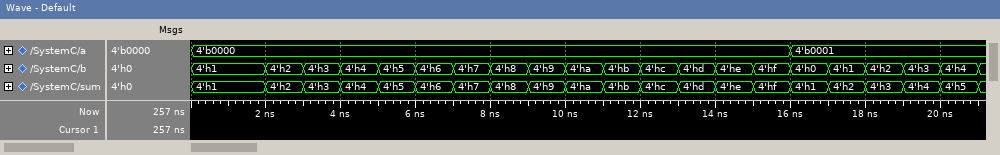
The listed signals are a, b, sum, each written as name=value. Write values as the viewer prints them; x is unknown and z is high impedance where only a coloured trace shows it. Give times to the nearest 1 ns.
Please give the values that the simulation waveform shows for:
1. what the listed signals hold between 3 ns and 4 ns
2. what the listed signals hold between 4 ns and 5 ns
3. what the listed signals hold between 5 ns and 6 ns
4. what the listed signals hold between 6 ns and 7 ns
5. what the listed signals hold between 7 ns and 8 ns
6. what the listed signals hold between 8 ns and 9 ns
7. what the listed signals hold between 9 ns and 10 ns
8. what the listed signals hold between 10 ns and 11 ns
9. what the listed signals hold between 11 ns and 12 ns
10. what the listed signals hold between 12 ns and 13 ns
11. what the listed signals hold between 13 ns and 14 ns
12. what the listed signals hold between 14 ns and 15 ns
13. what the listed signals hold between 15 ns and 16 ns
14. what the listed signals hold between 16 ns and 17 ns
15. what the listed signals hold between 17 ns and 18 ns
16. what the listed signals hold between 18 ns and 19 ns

a=4'b0000, b=4'h3, sum=4'h3
a=4'b0000, b=4'h4, sum=4'h4
a=4'b0000, b=4'h5, sum=4'h5
a=4'b0000, b=4'h6, sum=4'h6
a=4'b0000, b=4'h7, sum=4'h7
a=4'b0000, b=4'h8, sum=4'h8
a=4'b0000, b=4'h9, sum=4'h9
a=4'b0000, b=4'ha, sum=4'ha
a=4'b0000, b=4'hb, sum=4'hb
a=4'b0000, b=4'hc, sum=4'hc
a=4'b0000, b=4'hd, sum=4'hd
a=4'b0000, b=4'he, sum=4'he
a=4'b0000, b=4'hf, sum=4'hf
a=4'b0001, b=4'h0, sum=4'h1
a=4'b0001, b=4'h1, sum=4'h2
a=4'b0001, b=4'h2, sum=4'h3
